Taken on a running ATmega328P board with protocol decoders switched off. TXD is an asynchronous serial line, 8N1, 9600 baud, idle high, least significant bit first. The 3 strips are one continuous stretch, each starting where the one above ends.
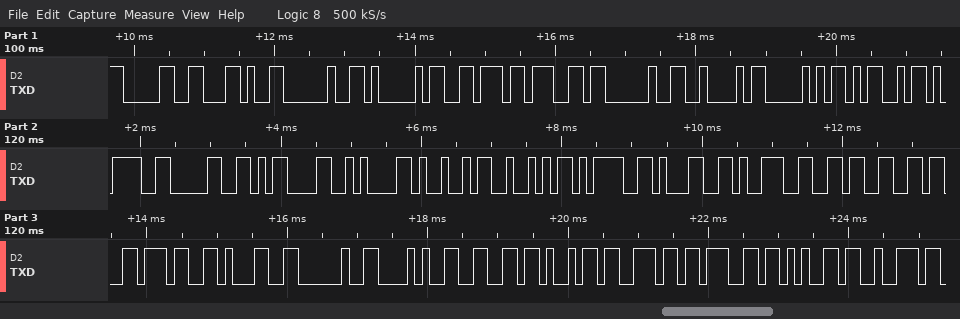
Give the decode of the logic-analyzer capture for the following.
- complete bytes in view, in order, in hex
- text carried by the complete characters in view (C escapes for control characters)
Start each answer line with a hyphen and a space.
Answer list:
- 30 2C 20 41 76 67 20 42 50 4D 3D 30 0D 0A 49 52 3D 31 39 36 36 37 31 20 28 66 69 6E 67 65 72
- "0, Avg BPM=0\r\nIR=196671 (finger"
